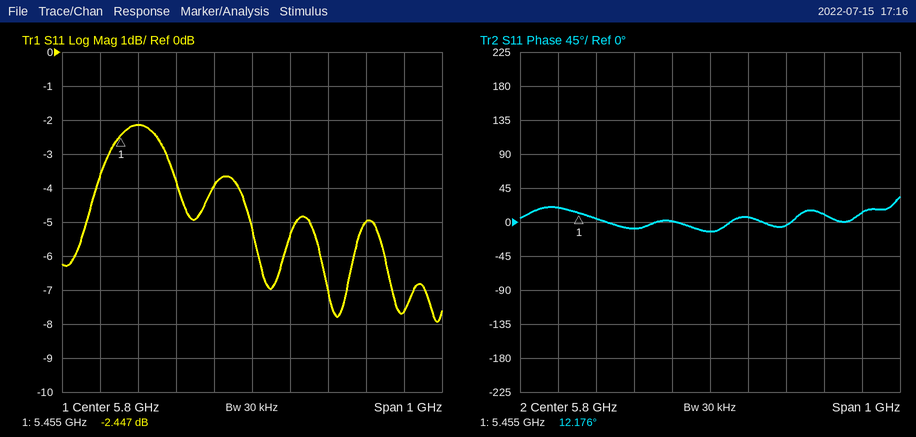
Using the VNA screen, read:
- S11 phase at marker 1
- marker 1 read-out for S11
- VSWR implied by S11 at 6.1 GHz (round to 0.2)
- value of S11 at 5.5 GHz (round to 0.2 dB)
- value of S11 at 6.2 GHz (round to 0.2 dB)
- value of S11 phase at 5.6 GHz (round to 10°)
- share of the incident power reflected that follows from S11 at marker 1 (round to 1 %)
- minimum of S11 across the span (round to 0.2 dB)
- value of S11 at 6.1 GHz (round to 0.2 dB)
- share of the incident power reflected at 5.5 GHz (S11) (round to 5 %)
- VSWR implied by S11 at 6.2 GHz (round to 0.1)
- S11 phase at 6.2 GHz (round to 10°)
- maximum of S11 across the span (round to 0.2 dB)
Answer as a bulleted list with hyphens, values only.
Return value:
- 12.176°
- -2.447 dB
- 3.6
- -2.2 dB
- -7.6 dB
- -10°
- 57 %
- -8.0 dB
- -5.0 dB
- 60 %
- 2.4
- 10°
- -2.2 dB
